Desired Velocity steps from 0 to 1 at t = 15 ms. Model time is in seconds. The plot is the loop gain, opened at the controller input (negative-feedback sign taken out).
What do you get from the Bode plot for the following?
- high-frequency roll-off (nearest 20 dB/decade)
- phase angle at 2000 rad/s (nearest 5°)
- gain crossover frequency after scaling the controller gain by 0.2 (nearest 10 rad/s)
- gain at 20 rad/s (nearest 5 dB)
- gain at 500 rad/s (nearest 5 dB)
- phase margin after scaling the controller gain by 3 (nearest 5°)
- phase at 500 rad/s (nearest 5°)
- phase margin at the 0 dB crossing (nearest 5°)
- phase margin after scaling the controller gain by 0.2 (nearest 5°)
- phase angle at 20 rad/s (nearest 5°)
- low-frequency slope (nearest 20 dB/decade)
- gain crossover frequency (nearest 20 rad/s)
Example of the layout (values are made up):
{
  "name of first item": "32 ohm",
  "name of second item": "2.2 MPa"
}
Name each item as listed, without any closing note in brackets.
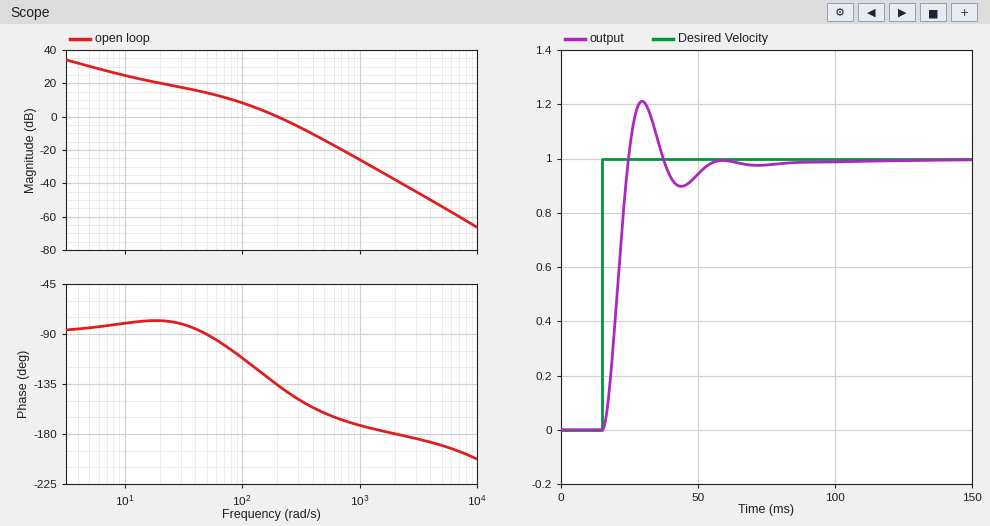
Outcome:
{
  "high-frequency roll-off": "-40 dB/decade",
  "phase angle at 2000 rad/s": "-180°",
  "gain crossover frequency after scaling the controller gain by 0.2": "50 rad/s",
  "gain at 20 rad/s": "20 dB",
  "gain at 500 rad/s": "-15 dB",
  "phase margin after scaling the controller gain by 3": "25°",
  "phase at 500 rad/s": "-160°",
  "phase margin at the 0 dB crossing": "45°",
  "phase margin after scaling the controller gain by 0.2": "90°",
  "phase angle at 20 rad/s": "-80°",
  "low-frequency slope": "-20 dB/decade",
  "gain crossover frequency": "200 rad/s"
}
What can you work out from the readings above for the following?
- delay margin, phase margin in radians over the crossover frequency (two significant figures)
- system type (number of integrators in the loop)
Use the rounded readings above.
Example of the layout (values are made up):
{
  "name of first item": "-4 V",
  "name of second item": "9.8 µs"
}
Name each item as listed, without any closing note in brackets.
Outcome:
{
  "delay margin, phase margin in radians over the crossover frequency": "0.0039 s",
  "system type": "1"
}
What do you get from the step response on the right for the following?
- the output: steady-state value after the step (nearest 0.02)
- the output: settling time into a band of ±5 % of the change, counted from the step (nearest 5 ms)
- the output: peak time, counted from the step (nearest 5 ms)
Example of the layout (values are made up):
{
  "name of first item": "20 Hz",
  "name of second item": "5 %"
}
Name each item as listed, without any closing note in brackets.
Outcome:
{
  "the output: steady-state value after the step": "1.00",
  "the output: settling time into a band of ±5 % of the change, counted from the step": "35 ms",
  "the output: peak time, counted from the step": "15 ms"
}
